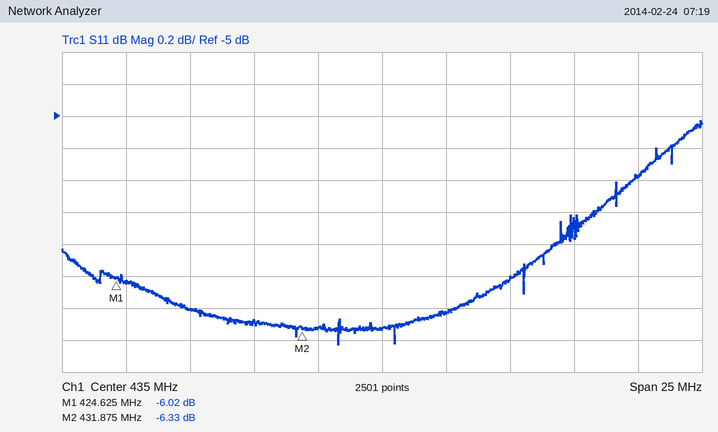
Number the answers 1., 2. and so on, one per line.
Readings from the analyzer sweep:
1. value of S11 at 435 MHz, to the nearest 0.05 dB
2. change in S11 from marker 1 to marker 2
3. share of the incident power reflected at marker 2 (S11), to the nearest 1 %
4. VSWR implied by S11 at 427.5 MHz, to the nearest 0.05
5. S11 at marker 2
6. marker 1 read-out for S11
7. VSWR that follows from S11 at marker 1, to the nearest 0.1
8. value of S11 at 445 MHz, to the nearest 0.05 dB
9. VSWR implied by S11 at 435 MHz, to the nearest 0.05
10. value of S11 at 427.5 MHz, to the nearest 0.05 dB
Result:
1. -6.35 dB
2. -0.31 dB
3. 23 %
4. 2.90
5. -6.33 dB
6. -6.02 dB
7. 3.0
8. -5.40 dB
9. 2.85
10. -6.20 dB
